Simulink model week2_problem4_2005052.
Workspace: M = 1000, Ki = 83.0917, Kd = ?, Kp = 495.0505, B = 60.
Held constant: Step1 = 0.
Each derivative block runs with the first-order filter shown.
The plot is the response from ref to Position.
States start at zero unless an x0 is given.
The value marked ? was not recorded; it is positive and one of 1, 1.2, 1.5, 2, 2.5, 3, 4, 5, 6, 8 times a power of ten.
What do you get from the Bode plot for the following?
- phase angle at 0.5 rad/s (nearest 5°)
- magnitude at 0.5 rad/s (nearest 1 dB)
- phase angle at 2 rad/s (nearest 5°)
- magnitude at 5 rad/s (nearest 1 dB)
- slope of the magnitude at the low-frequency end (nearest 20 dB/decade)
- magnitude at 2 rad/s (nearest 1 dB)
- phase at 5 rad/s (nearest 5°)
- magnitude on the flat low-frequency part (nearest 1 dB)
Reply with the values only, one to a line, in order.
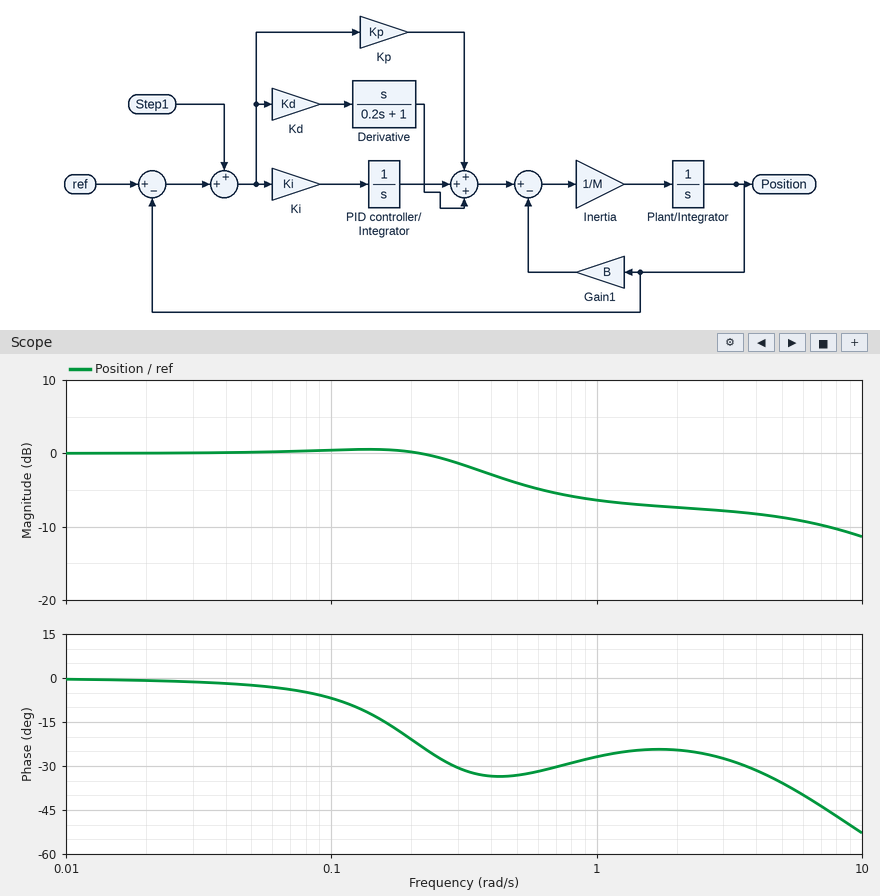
-35°
-4 dB
-25°
-9 dB
0 dB/decade
-7 dB
-35°
0 dB
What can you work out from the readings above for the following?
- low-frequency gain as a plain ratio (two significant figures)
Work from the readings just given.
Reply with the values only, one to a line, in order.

1.0
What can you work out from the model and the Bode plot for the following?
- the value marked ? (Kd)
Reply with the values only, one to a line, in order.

600
